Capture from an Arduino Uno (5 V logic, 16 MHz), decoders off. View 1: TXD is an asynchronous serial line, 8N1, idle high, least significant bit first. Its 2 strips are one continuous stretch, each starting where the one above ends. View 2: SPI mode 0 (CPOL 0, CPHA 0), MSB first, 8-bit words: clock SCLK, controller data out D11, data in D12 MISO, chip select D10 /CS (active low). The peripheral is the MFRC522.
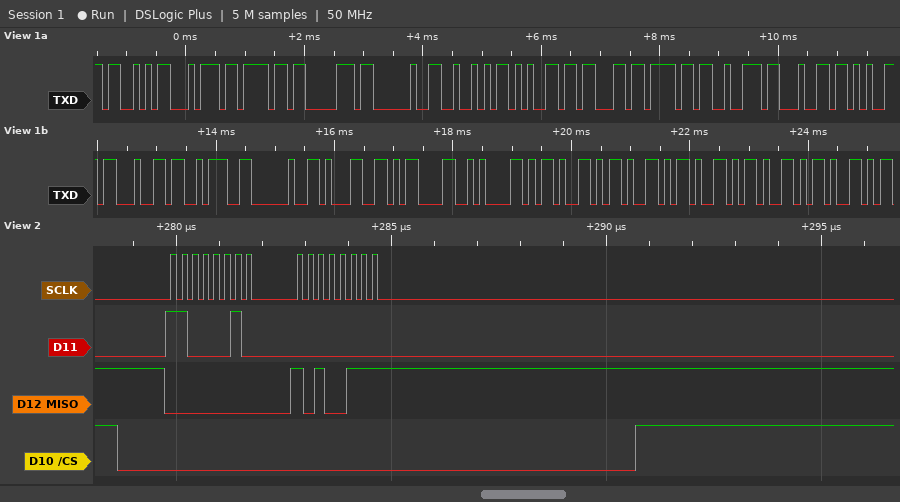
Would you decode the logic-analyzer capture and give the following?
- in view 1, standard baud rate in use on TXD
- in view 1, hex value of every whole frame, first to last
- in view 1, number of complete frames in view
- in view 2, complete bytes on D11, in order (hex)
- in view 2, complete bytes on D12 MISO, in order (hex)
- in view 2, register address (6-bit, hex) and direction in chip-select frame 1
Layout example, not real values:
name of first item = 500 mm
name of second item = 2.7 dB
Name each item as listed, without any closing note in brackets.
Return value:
in view 1, standard baud rate in use on TXD = 9600 baud
in view 1, hex value of every whole frame, first to last = 53 74 6F 70 20 52 65 63 6F 72 64 65 64 3A 20 31 0D 0A 2D 2D 2D 2D 2D
in view 1, number of complete frames in view = 23
in view 2, complete bytes on D11, in order = C2 00
in view 2, complete bytes on D12 MISO, in order = 00 A7
in view 2, register address (6-bit, hex) and direction in chip-select frame 1 = 0x21 read
